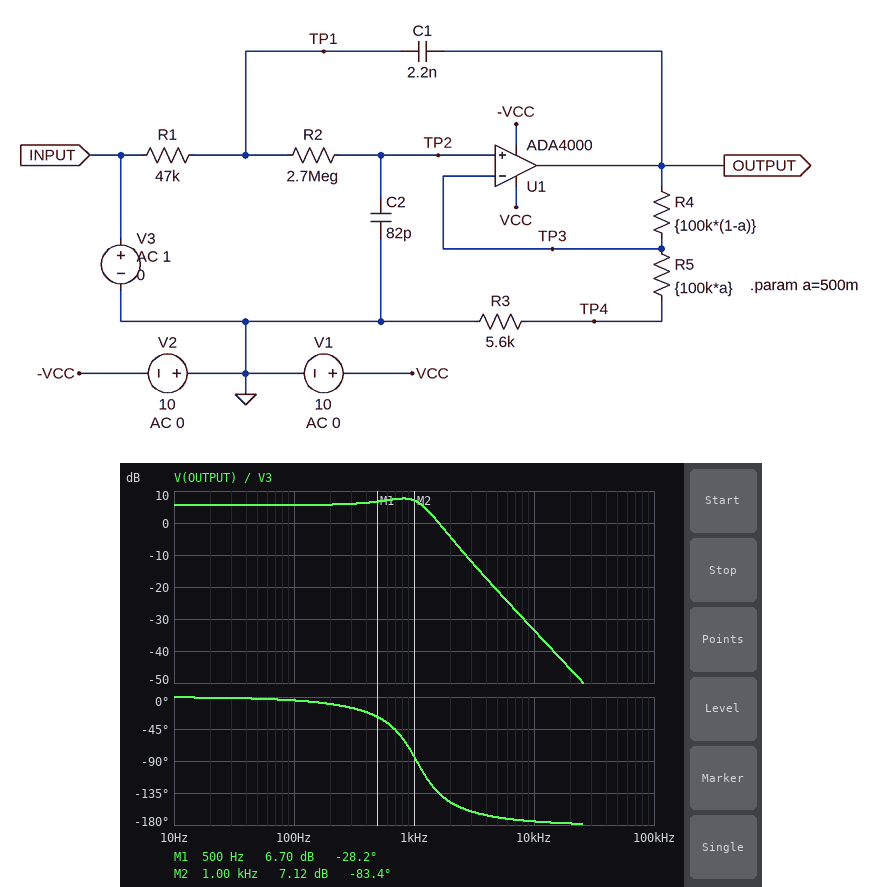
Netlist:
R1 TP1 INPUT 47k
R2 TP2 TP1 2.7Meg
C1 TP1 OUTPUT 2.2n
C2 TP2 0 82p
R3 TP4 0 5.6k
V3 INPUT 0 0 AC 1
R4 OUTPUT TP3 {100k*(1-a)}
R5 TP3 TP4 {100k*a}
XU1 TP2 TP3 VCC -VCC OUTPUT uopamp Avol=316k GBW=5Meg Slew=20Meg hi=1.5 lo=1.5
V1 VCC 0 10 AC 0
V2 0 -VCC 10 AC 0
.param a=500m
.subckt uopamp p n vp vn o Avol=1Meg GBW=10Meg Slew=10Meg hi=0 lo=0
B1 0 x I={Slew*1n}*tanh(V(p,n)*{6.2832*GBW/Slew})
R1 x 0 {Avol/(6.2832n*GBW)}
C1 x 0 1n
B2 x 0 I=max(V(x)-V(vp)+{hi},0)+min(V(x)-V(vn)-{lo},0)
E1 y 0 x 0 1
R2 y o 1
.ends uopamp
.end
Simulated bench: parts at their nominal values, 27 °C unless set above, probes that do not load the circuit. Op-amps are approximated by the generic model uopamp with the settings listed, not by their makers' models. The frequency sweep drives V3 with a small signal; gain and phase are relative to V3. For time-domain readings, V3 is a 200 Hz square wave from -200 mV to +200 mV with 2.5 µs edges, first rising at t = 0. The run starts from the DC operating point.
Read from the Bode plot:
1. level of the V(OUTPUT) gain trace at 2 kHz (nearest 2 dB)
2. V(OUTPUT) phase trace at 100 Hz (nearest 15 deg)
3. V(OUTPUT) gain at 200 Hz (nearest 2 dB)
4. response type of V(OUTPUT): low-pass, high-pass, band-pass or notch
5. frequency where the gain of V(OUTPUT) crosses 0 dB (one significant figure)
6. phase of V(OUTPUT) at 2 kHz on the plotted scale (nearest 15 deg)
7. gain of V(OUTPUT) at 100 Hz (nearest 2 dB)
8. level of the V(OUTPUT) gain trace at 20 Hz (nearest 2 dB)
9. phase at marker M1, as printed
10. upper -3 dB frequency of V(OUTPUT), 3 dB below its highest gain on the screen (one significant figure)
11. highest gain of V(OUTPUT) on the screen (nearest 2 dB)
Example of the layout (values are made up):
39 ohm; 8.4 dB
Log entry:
-4 dB; 0 deg; 6 dB; low-pass; 2 kHz; -150 deg; 6 dB; 6 dB; -28.2 deg; 1 kHz; 8 dB
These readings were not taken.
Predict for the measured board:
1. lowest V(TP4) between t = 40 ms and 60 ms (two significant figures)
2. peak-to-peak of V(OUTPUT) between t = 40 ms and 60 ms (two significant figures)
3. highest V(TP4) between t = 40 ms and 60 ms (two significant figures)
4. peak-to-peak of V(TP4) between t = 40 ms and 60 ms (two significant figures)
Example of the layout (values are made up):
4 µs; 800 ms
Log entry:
-29 mV; 1.1 V; 29 mV; 58 mV
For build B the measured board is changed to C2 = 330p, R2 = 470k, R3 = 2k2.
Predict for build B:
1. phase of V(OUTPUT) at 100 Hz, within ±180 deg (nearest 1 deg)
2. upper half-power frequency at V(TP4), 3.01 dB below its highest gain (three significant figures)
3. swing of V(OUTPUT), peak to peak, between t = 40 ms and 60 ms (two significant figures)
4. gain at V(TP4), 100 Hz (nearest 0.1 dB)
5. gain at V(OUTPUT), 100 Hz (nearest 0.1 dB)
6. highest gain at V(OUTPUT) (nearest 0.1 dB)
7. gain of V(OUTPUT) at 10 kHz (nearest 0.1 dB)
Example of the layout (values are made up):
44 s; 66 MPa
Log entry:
-3 deg; 1.48 kHz; 1.4 V; -27.5 dB; 5.9 dB; 11.2 dB; -30.1 dB
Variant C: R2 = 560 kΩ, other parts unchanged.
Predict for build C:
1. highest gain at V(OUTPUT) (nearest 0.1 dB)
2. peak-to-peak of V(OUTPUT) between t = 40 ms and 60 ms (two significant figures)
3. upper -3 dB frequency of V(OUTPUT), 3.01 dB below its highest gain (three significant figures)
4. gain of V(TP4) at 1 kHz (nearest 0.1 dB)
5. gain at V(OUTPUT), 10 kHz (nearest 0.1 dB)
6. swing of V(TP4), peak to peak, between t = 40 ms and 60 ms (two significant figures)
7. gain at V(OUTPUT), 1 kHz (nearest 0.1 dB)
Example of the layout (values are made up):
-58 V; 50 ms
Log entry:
10.1 dB; 17 V; 2.73 kHz; -18.6 dB; -19.5 dB; 900 mV; 6.9 dB
